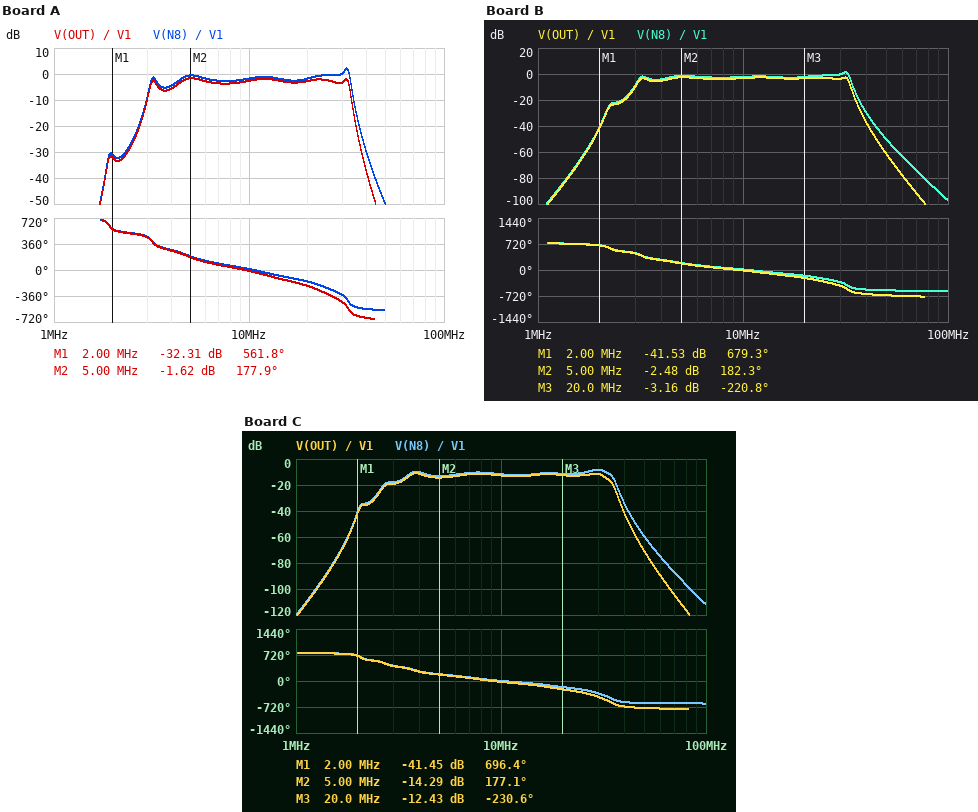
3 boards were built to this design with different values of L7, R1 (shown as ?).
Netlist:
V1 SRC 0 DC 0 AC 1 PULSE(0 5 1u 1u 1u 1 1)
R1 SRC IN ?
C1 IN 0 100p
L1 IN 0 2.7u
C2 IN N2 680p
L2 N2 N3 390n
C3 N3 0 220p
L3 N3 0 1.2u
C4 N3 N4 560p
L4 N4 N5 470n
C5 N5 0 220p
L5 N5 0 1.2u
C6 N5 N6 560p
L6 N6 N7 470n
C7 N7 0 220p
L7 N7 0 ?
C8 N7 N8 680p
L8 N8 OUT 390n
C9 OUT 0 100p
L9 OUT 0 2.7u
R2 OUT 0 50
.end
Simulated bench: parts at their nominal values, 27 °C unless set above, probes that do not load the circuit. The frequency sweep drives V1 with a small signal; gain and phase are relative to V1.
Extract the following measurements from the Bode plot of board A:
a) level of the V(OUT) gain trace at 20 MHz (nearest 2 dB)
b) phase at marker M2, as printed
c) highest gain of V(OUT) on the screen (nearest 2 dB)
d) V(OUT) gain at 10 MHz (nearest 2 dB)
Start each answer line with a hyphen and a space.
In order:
- -2 dB
- 177.9 deg
- -2 dB
- -2 dB
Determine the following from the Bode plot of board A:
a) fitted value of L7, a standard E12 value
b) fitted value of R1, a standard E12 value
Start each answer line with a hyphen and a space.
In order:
- 3.9 µH
- 18 Ω
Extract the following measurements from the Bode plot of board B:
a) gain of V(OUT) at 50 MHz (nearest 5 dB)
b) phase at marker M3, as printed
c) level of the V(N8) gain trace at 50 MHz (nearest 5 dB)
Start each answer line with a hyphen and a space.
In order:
- -60 dB
- -220.8 deg
- -50 dB
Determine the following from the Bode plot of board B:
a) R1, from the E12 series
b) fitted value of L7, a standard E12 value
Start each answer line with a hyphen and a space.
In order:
- 22 Ω
- 2.7 µH
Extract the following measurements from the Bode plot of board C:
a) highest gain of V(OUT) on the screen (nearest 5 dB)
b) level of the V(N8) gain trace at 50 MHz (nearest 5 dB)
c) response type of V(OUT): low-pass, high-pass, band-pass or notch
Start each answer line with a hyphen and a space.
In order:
- -10 dB
- -60 dB
- band-pass
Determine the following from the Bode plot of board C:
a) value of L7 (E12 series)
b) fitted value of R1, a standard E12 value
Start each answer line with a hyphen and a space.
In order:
- 3.3 µH
- 150 Ω
